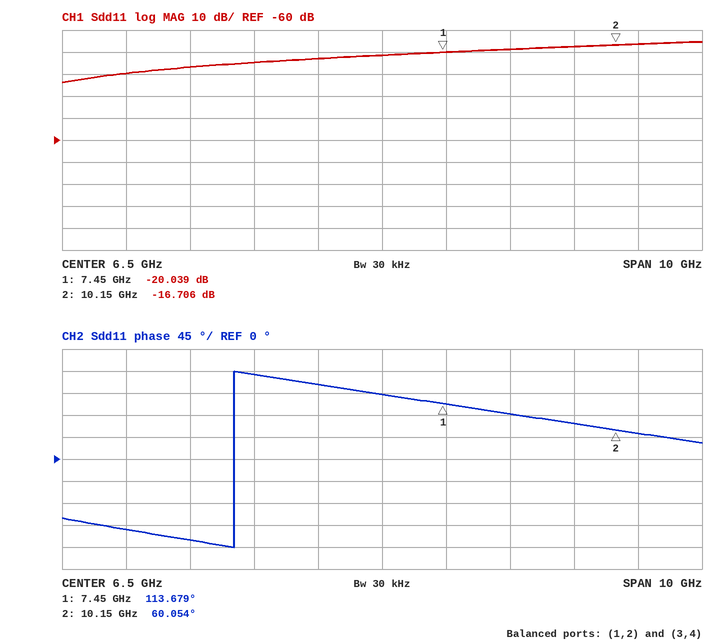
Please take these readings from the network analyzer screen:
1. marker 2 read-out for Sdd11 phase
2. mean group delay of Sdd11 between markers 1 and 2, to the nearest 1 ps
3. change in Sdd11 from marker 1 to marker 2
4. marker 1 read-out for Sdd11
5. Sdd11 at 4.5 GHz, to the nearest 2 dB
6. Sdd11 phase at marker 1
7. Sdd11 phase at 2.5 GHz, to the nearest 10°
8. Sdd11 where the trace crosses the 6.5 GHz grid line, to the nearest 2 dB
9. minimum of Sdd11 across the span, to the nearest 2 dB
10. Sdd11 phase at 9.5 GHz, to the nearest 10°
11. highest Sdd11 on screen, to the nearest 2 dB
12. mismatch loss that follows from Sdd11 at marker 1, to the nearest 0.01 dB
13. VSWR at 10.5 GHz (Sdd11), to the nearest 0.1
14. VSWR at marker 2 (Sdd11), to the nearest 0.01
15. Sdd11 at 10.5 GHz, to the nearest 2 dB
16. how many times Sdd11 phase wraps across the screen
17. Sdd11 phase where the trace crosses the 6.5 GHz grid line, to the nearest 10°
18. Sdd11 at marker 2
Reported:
60.054°
55 ps
3.333 dB
-20.039 dB
-24 dB
113.679°
-140°
-22 dB
-34 dB
70°
-16 dB
0.04 dB
1.4
1.34
-16 dB
1
130°
-16.706 dB
